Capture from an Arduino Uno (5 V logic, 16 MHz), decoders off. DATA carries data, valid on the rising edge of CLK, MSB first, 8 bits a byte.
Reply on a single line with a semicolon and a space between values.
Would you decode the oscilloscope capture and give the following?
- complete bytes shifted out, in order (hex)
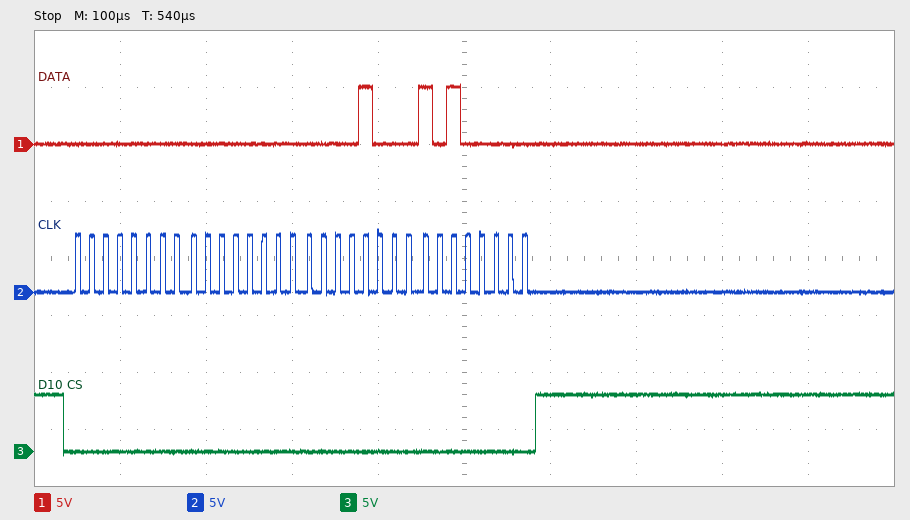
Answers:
0x00 0x00 0x08 0xA0
